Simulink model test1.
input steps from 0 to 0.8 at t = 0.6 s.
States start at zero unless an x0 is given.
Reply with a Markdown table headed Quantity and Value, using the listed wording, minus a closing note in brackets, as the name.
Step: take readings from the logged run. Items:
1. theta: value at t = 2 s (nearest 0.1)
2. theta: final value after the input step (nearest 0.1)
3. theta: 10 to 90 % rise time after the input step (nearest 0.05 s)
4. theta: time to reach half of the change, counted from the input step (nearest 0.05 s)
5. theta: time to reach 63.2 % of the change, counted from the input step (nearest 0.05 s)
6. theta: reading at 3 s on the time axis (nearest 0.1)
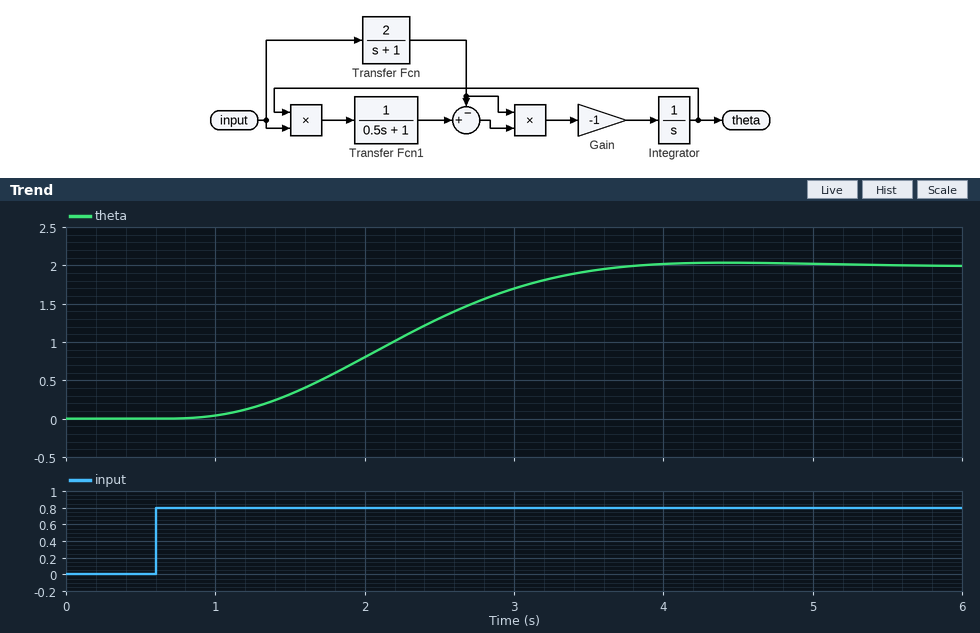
| Quantity | Value |
|---|---|
| theta: value at t = 2 s | 0.8 |
| theta: final value after the input step | 2.0 |
| theta: 10 to 90 % rise time after the input step | 1.85 s |
| theta: time to reach half of the change, counted from the input step | 1.60 s |
| theta: time to reach 63.2 % of the change, counted from the input step | 1.85 s |
| theta: reading at 3 s on the time axis | 1.7 |
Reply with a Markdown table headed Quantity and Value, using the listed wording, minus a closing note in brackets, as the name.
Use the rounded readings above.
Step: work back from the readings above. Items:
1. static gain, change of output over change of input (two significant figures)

| Quantity | Value |
|---|---|
| static gain, change of output over change of input | 2.5 |
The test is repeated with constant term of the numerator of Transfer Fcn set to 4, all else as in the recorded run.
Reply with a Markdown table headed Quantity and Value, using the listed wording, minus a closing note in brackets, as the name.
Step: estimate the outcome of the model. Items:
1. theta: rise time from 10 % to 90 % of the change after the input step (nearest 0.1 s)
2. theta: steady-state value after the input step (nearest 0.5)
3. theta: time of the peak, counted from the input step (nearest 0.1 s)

| Quantity | Value |
|---|---|
| theta: rise time from 10 % to 90 % of the change after the input step | 1.2 s |
| theta: steady-state value after the input step | 4.0 |
| theta: time of the peak, counted from the input step | 2.4 s |
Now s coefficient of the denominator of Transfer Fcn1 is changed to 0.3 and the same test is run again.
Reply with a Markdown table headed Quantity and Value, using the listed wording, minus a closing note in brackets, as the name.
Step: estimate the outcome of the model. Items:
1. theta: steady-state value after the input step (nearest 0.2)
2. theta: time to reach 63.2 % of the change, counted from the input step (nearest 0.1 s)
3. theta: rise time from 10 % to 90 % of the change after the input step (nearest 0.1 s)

| Quantity | Value |
|---|---|
| theta: steady-state value after the input step | 2.0 |
| theta: time to reach 63.2 % of the change, counted from the input step | 2.0 s |
| theta: rise time from 10 % to 90 % of the change after the input step | 2.3 s |
